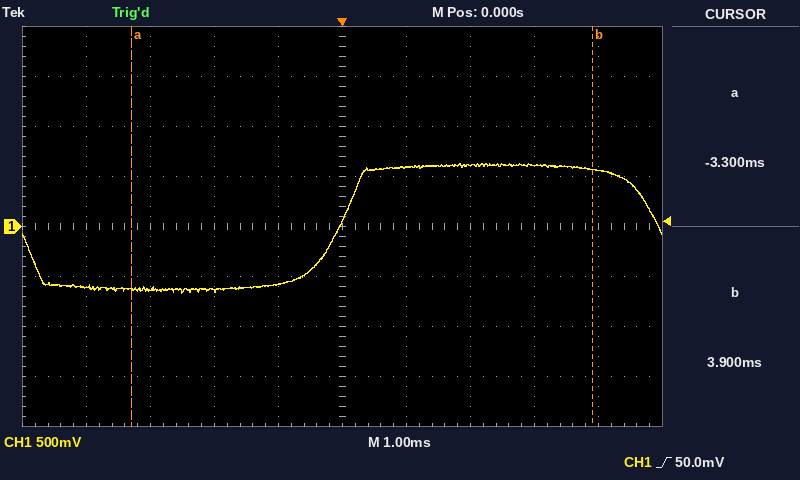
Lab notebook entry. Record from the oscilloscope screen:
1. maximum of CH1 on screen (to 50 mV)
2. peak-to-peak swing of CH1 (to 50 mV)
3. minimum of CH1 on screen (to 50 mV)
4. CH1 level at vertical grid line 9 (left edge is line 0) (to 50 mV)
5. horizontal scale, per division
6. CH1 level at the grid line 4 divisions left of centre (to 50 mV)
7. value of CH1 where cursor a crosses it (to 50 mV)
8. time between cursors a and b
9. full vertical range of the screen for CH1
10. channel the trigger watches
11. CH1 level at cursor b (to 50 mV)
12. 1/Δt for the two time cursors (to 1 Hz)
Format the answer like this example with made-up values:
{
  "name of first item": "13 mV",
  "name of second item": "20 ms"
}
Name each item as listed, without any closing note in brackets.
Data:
{
  "maximum of CH1 on screen": "650 mV",
  "peak-to-peak swing of CH1": "1.30 V",
  "minimum of CH1 on screen": "-650 mV",
  "CH1 level at vertical grid line 9 (left edge is line 0)": "550 mV",
  "horizontal scale, per division": "1 ms",
  "CH1 level at the grid line 4 divisions left of centre": "-600 mV",
  "value of CH1 where cursor a crosses it": "-650 mV",
  "time between cursors a and b": "7.2 ms",
  "full vertical range of the screen for CH1": "4 V",
  "channel the trigger watches": "CH1",
  "CH1 level at cursor b": "550 mV",
  "1/Δt for the two time cursors": "139 Hz"
}
